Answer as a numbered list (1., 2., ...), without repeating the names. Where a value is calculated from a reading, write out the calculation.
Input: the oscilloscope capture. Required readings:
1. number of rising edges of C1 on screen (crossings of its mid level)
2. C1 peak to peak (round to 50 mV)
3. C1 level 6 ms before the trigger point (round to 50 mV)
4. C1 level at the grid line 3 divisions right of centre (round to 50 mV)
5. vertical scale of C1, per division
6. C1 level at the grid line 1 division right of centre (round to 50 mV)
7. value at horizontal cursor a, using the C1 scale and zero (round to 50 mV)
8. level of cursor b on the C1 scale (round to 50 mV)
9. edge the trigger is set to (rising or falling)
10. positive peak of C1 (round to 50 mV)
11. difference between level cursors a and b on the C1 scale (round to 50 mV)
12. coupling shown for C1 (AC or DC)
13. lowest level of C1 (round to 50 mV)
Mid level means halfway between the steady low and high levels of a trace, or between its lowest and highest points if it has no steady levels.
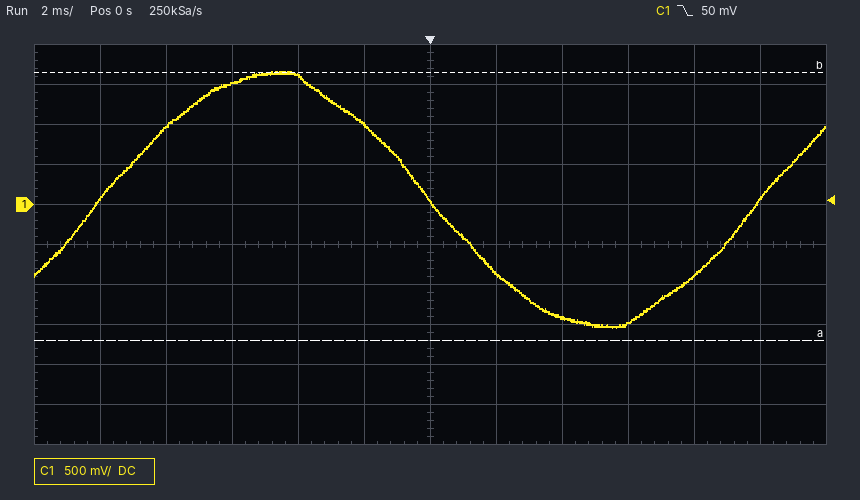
1. 2
2. 1.65 V − (-1.55 V) = 3.20 V
3. 1.50 V
4. -1.50 V
5. 500 mV
6. -850 mV
7. -1.70 V
8. 1.65 V
9. falling
10. 1.65 V
11. 3.35 V
12. DC
13. -1.55 V
